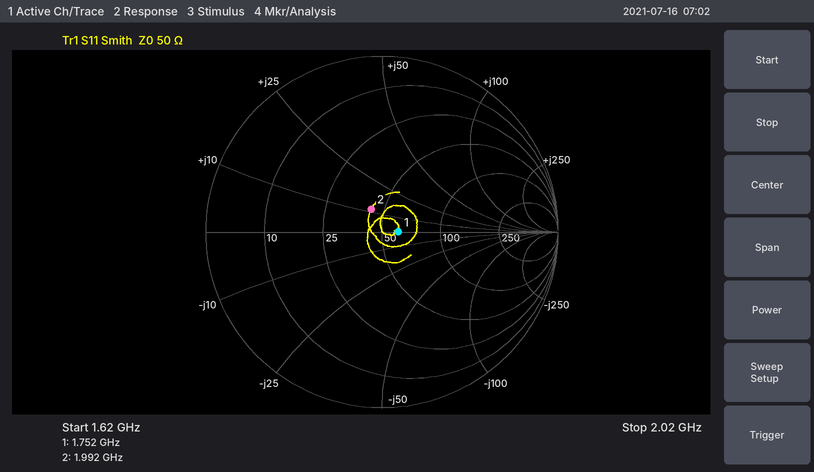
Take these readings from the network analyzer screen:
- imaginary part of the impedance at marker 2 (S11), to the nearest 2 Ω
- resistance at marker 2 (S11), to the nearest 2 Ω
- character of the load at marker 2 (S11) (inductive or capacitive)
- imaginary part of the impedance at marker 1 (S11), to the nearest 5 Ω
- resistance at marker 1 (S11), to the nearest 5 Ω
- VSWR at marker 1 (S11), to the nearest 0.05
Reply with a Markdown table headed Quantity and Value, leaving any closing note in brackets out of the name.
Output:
| Quantity | Value |
|---|---|
| imaginary part of the impedance at marker 2 (S11), to the nearest 2 Ω | +12 Ω |
| resistance at marker 2 (S11), to the nearest 2 Ω | 42 Ω |
| character of the load at marker 2 (S11) | inductive |
| imaginary part of the impedance at marker 1 (S11), to the nearest 5 Ω | 0 Ω |
| resistance at marker 1 (S11), to the nearest 5 Ω | 60 Ω |
| VSWR at marker 1 (S11), to the nearest 0.05 | 1.20 |
